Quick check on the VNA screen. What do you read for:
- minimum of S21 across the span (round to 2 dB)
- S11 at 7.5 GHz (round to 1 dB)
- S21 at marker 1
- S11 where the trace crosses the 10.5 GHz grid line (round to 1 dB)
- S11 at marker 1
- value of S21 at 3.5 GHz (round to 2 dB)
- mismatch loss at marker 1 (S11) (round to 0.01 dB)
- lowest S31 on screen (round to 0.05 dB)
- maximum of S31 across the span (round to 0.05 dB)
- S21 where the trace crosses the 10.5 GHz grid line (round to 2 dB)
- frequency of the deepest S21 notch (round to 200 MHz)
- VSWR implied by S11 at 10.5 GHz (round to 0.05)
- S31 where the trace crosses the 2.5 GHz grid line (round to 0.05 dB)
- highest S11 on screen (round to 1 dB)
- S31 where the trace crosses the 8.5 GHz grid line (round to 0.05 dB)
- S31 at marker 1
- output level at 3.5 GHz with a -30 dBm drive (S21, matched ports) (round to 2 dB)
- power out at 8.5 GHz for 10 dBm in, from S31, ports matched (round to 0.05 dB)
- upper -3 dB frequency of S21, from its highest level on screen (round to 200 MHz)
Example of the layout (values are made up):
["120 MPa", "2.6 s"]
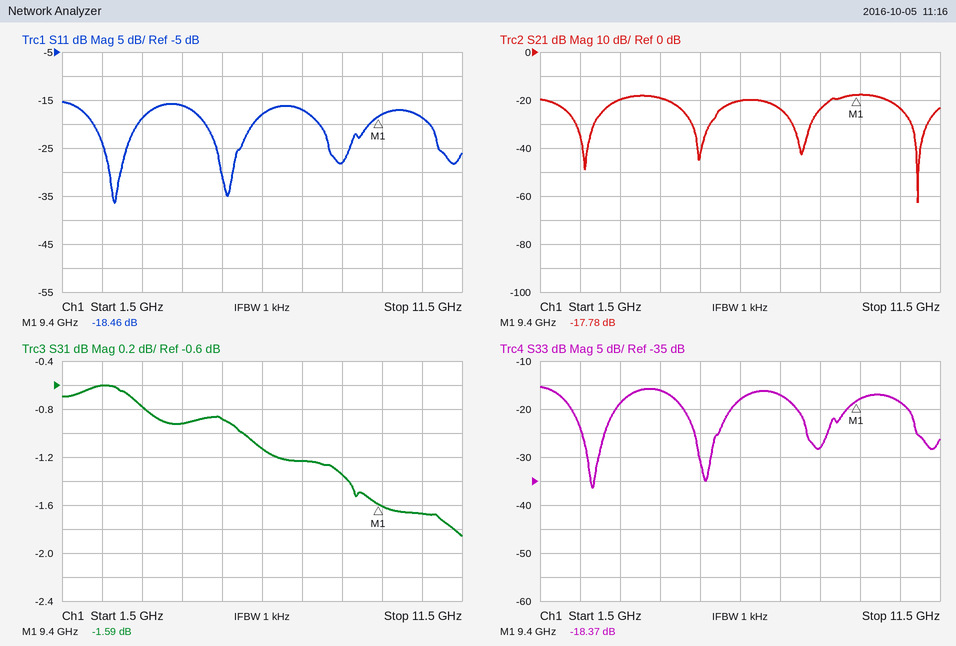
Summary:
["-62 dB", "-17 dB", "-17.78 dB", "-19 dB", "-18.46 dB", "-20 dB", "0.06 dB", "-1.85 dB", "-0.60 dB", "-24 dB", "11.0 GHz", "1.25", "-0.60 dB", "-15 dB", "-1.35 dB", "-1.59 dB", "-50 dBm", "8.65 dBm", "10.2 GHz"]
